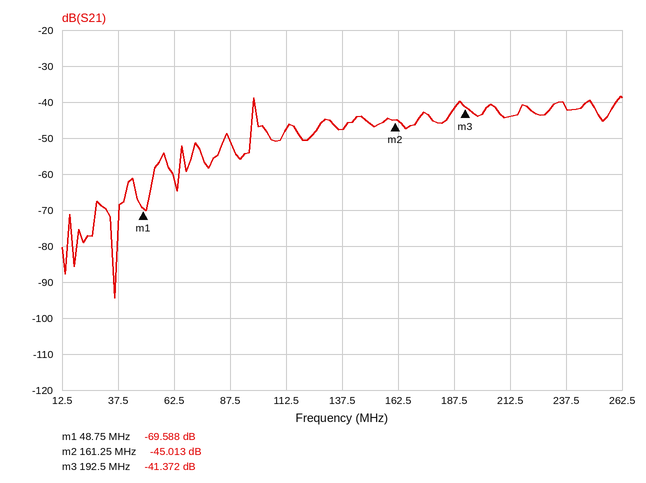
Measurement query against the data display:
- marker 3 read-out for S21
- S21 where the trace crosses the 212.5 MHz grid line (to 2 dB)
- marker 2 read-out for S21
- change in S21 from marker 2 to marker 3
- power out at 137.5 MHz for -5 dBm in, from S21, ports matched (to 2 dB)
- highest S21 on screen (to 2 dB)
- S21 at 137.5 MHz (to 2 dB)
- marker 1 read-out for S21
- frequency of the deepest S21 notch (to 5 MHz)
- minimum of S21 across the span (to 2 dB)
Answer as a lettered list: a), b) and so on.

a) -41.372 dB
b) -44 dB
c) -45.013 dB
d) 3.641 dB
e) -52 dBm
f) -38 dB
g) -48 dB
h) -69.588 dB
i) 35 MHz
j) -94 dB
